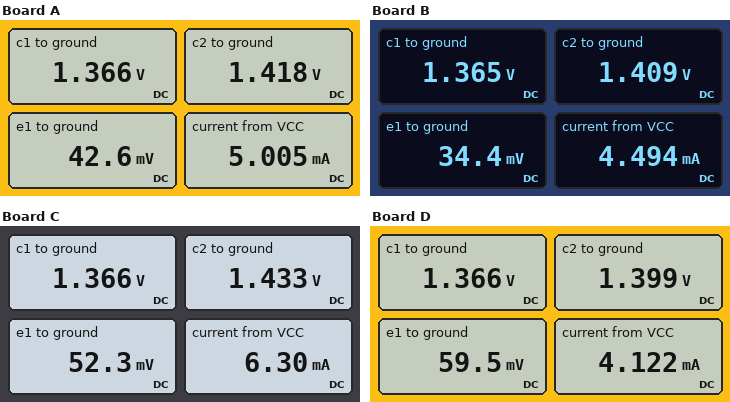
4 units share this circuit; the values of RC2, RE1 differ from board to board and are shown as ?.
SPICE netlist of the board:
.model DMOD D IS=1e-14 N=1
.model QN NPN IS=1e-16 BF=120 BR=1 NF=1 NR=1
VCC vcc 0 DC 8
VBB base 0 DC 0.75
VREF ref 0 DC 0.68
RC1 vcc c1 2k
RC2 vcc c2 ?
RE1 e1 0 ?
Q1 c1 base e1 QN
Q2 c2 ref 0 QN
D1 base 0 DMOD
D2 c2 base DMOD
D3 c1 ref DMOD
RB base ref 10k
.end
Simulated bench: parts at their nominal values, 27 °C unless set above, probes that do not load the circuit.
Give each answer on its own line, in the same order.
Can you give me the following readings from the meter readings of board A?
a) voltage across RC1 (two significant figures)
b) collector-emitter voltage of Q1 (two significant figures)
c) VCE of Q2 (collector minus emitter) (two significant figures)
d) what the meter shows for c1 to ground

6.6 V
1.3 V
1.4 V
1.366 V
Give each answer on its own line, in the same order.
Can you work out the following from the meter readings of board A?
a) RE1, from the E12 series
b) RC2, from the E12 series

560 Ω
3.9 kΩ
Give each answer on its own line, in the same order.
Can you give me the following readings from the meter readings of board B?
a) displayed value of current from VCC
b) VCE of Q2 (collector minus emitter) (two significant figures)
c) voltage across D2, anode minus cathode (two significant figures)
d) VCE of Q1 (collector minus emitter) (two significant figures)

4.494 mA
1.4 V
660 mV
1.3 V
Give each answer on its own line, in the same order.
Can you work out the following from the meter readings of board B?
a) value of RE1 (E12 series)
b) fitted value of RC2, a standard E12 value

330 Ω
5.6 kΩ
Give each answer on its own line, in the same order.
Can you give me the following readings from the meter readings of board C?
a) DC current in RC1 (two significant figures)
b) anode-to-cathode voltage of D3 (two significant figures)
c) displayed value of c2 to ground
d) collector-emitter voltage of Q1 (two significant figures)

3.3 mA
690 mV
1.433 V
1.3 V
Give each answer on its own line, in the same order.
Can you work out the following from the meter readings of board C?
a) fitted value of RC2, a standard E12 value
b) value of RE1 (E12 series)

2.2 kΩ
1 kΩ
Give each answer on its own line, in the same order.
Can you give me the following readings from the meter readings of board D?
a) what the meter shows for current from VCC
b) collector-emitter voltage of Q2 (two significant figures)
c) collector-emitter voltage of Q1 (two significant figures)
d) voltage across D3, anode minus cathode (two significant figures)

4.122 mA
1.4 V
1.3 V
690 mV
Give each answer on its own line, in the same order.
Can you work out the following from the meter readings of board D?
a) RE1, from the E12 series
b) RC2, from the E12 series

1.5 kΩ
8.2 kΩ
